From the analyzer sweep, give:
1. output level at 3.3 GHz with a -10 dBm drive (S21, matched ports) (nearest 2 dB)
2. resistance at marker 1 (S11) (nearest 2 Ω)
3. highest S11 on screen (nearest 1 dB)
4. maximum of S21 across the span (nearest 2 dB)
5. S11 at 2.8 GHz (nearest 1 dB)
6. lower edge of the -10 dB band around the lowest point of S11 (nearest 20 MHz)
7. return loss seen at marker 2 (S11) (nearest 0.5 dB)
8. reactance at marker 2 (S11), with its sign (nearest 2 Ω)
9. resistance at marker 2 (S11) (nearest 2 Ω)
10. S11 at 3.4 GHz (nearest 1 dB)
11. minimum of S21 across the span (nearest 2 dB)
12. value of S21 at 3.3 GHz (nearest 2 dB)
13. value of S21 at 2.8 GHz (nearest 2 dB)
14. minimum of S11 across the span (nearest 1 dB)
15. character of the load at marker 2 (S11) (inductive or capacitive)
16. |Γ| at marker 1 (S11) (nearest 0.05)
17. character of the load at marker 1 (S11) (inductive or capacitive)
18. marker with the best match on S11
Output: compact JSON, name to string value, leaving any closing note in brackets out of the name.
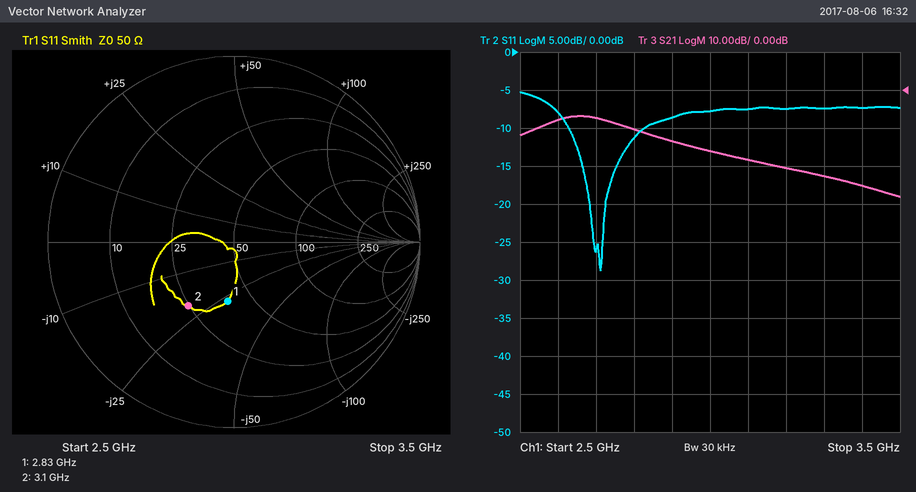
{"output level at 3.3 GHz with a -10 dBm drive (S21, matched ports)": "-32 dBm", "resistance at marker 1 (S11)": "38 Ω", "highest S11 on screen": "-5 dB", "maximum of S21 across the span": "-6 dB", "S11 at 2.8 GHz": "-11 dB", "lower edge of the -10 dB band around the lowest point of S11": "2.62 GHz", "return loss seen at marker 2 (S11)": "7.5 dB", "reactance at marker 2 (S11), with its sign": "-20 Ω", "resistance at marker 2 (S11)": "24 Ω", "S11 at 3.4 GHz": "-7 dB", "minimum of S21 across the span": "-28 dB", "value of S21 at 3.3 GHz": "-22 dB", "value of S21 at 2.8 GHz": "-10 dB", "minimum of S11 across the span": "-29 dB", "character of the load at marker 2 (S11)": "capacitive", "|Γ| at marker 1 (S11)": "0.30", "character of the load at marker 1 (S11)": "capacitive", "marker with the best match on S11": "marker 1"}
